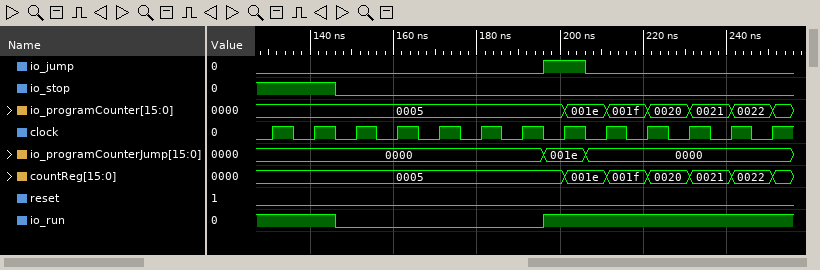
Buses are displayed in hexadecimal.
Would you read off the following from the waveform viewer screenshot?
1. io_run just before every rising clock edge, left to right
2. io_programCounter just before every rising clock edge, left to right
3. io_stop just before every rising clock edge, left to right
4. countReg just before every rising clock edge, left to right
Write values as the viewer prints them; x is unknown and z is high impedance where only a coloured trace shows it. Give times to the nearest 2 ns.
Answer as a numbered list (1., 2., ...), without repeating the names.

1. 1 1 0 0 0 0 0 1 1 1 1 1 1
2. 0005, 0005, 0005, 0005, 0005, 0005, 0005, 0005, 001e, 001f, 0020, 0021, 0022
3. 1 1 0 0 0 0 0 0 0 0 0 0 0
4. 0005, 0005, 0005, 0005, 0005, 0005, 0005, 0005, 001e, 001f, 0020, 0021, 0022
